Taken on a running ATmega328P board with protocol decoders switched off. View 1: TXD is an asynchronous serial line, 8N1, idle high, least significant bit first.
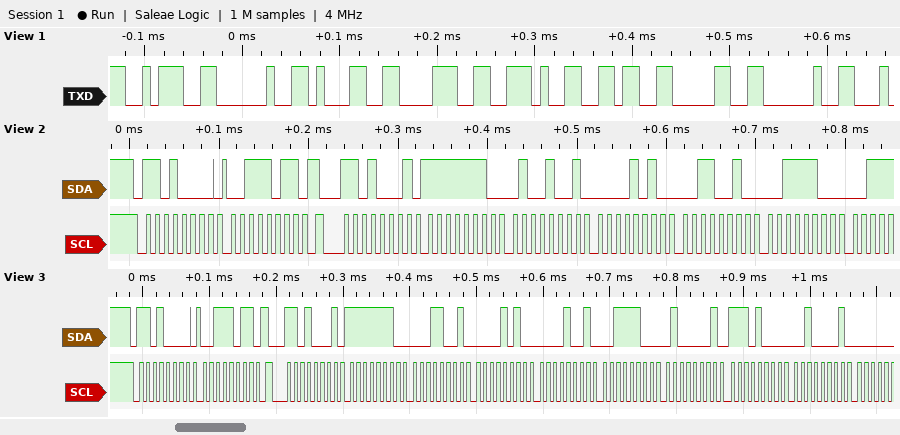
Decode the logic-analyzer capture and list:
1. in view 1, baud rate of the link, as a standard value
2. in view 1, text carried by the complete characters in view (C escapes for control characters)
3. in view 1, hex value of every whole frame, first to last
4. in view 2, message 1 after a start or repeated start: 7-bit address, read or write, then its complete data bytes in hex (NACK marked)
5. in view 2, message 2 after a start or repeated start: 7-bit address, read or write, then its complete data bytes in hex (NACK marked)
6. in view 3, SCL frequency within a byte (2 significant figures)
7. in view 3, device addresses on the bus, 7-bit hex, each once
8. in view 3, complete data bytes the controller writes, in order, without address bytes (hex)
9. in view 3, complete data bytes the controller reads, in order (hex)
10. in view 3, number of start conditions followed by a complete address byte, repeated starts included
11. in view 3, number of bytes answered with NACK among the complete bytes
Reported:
115200 baud
": 18.60 "
3A 20 31 38 2E 36 30 20
0x68 write: 3B
0x68 read: FE 49 0A 32 3C
100 kHz
0x68
3B
FE 19 0A 09 3C 41 E8 21
2
0
